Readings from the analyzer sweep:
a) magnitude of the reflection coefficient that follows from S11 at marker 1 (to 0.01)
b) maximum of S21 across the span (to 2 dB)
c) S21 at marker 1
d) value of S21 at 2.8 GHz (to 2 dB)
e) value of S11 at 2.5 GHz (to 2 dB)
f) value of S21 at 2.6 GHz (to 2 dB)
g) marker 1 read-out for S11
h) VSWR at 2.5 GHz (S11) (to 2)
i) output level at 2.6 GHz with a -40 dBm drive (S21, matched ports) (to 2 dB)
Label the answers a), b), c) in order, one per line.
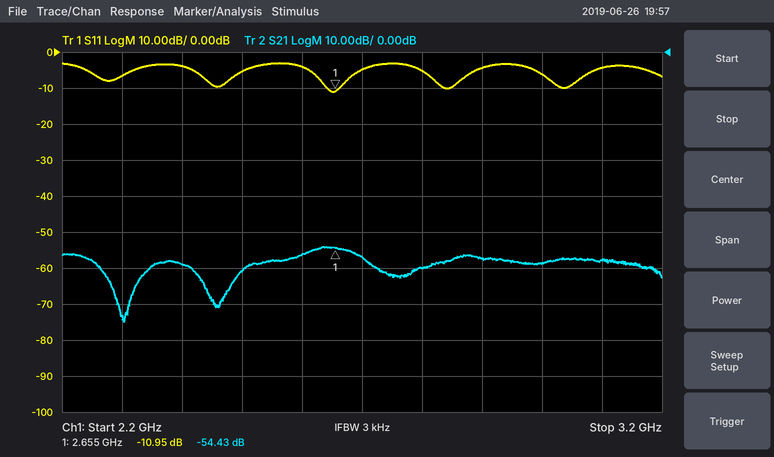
a) 0.28
b) -54 dB
c) -54.43 dB
d) -60 dB
e) -6 dB
f) -56 dB
g) -10.95 dB
h) 4
i) -96 dBm
